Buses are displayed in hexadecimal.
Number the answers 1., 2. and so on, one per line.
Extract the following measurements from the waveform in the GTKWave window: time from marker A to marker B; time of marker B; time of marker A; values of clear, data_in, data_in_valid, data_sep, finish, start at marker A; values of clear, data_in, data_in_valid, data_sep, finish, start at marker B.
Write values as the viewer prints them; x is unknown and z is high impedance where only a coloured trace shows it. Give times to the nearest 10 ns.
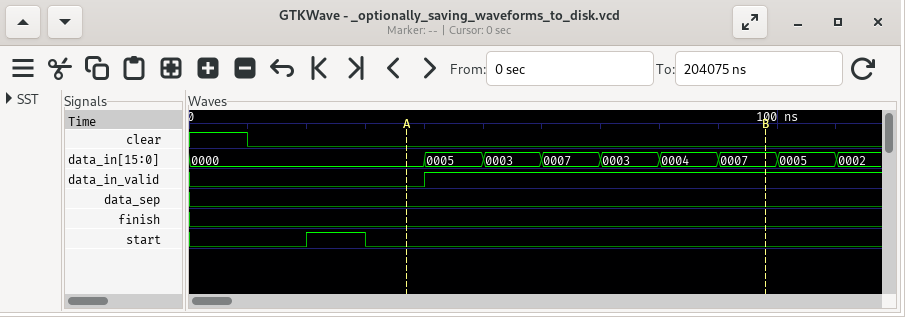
1. 60 ns
2. 100 ns
3. 40 ns
4. clear=0, data_in=0000, data_in_valid=0, data_sep=0, finish=0, start=0
5. clear=0, data_in=0007, data_in_valid=1, data_sep=0, finish=0, start=0
